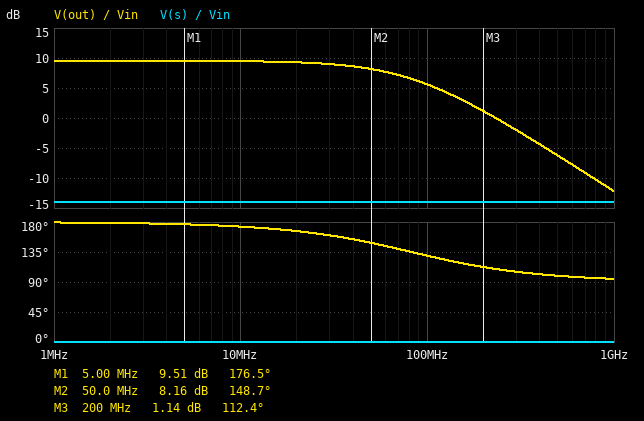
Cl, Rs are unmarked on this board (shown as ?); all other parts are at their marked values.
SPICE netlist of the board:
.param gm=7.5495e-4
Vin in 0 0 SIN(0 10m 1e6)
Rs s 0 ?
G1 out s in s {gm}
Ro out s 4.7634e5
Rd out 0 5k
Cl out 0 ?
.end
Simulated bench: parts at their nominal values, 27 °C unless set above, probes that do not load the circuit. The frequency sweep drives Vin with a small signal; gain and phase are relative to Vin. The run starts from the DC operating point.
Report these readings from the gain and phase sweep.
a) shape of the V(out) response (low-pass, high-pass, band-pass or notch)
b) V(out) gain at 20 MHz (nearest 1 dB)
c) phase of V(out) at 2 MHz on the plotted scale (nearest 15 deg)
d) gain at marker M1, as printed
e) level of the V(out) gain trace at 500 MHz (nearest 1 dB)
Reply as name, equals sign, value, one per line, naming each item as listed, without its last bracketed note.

shape of the V(out) response = low-pass
V(out) gain at 20 MHz = 9 dB
phase of V(out) at 2 MHz on the plotted scale = 180 deg
gain at marker M1, as printed = 9.51 dB
level of the V(out) gain trace at 500 MHz = -6 dB
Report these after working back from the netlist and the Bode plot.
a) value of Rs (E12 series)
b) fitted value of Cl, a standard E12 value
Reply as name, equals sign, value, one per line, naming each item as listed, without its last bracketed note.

value of Rs = 330 Ω
fitted value of Cl, a standard E12 value = 390 fF
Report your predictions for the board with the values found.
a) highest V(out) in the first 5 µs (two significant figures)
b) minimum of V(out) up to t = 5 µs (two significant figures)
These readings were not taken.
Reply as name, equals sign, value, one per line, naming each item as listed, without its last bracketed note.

highest V(out) in the first 5 µs = 30 mV
minimum of V(out) up to t = 5 µs = -30 mV
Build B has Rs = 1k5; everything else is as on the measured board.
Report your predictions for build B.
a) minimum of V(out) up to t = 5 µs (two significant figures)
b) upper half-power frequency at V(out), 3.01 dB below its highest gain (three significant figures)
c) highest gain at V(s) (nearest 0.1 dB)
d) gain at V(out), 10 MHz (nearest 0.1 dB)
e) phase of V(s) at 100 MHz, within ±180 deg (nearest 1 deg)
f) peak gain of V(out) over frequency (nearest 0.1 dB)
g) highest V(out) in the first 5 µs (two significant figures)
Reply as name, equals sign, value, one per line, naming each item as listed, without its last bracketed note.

minimum of V(out) up to t = 5 µs = -18 mV
upper half-power frequency at V(out), 3.01 dB below its highest gain = 82.0 MHz
highest gain at V(s) = -5.5 dB
gain at V(out), 10 MHz = 4.8 dB
phase of V(s) at 100 MHz, within ±180 deg = 0 deg
peak gain of V(out) over frequency = 4.9 dB
highest V(out) in the first 5 µs = 18 mV
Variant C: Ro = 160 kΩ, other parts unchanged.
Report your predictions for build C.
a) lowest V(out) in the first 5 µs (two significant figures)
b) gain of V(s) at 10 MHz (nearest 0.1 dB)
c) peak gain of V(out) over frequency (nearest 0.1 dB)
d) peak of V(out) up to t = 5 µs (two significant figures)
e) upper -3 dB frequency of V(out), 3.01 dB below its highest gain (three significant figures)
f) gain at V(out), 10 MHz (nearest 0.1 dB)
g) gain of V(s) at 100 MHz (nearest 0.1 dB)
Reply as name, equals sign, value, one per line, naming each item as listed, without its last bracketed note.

lowest V(out) in the first 5 µs = -29 mV
gain of V(s) at 10 MHz = -14.2 dB
peak gain of V(out) over frequency = 9.4 dB
peak of V(out) up to t = 5 µs = 29 mV
upper -3 dB frequency of V(out), 3.01 dB below its highest gain = 83.7 MHz
gain at V(out), 10 MHz = 9.3 dB
gain of V(s) at 100 MHz = -14.1 dB
